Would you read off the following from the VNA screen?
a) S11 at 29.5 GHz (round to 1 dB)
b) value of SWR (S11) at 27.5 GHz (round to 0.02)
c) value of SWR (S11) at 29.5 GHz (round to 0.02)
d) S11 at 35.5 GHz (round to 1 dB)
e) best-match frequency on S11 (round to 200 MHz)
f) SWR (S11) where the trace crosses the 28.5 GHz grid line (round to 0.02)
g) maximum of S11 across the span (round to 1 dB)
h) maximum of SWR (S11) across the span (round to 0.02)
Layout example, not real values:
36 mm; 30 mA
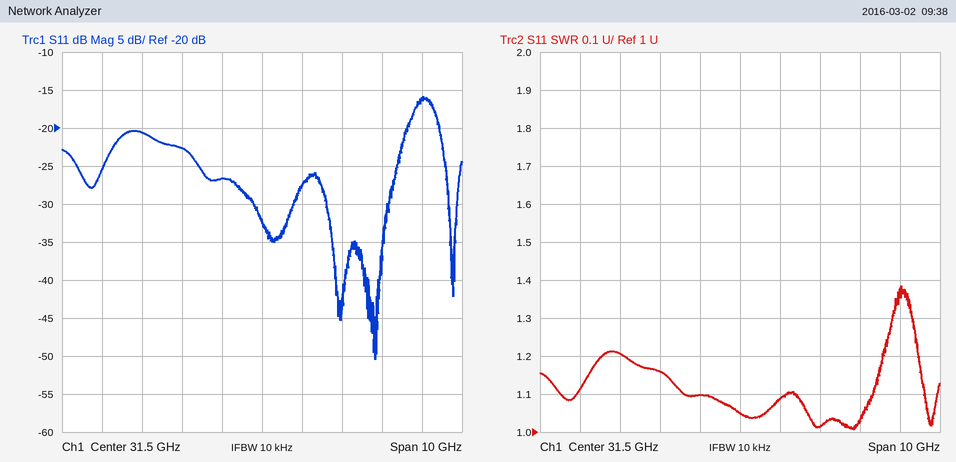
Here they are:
-23 dB; 1.12; 1.16; -16 dB; 34.4 GHz; 1.20; -16 dB; 1.38
